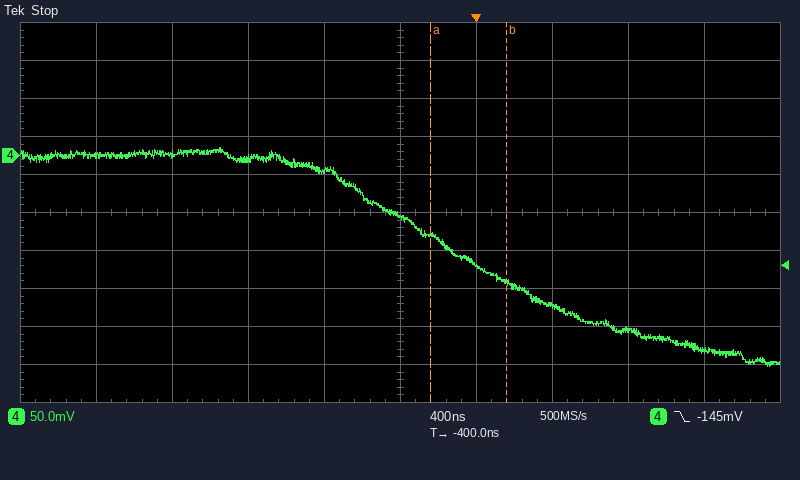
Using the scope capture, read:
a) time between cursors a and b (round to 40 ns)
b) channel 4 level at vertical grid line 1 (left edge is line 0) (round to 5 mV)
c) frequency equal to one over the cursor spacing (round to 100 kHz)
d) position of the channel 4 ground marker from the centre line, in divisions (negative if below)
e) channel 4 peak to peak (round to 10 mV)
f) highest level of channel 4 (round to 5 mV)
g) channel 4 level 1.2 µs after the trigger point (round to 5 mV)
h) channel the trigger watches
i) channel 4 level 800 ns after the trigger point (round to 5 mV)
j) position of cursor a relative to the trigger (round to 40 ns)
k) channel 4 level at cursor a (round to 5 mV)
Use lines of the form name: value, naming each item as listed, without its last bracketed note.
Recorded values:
time between cursors a and b: 400 ns
channel 4 level at vertical grid line 1 (left edge is line 0): 0 mV
frequency equal to one over the cursor spacing: 2.5 MHz
position of the channel 4 ground marker from the centre line, in divisions: +1.5 div
channel 4 peak to peak: 290 mV
highest level of channel 4: 10 mV
channel 4 level 1.2 µs after the trigger point: -255 mV
channel the trigger watches: channel 4
channel 4 level 800 ns after the trigger point: -230 mV
position of cursor a relative to the trigger: -240 ns
channel 4 level at cursor a: -105 mV
